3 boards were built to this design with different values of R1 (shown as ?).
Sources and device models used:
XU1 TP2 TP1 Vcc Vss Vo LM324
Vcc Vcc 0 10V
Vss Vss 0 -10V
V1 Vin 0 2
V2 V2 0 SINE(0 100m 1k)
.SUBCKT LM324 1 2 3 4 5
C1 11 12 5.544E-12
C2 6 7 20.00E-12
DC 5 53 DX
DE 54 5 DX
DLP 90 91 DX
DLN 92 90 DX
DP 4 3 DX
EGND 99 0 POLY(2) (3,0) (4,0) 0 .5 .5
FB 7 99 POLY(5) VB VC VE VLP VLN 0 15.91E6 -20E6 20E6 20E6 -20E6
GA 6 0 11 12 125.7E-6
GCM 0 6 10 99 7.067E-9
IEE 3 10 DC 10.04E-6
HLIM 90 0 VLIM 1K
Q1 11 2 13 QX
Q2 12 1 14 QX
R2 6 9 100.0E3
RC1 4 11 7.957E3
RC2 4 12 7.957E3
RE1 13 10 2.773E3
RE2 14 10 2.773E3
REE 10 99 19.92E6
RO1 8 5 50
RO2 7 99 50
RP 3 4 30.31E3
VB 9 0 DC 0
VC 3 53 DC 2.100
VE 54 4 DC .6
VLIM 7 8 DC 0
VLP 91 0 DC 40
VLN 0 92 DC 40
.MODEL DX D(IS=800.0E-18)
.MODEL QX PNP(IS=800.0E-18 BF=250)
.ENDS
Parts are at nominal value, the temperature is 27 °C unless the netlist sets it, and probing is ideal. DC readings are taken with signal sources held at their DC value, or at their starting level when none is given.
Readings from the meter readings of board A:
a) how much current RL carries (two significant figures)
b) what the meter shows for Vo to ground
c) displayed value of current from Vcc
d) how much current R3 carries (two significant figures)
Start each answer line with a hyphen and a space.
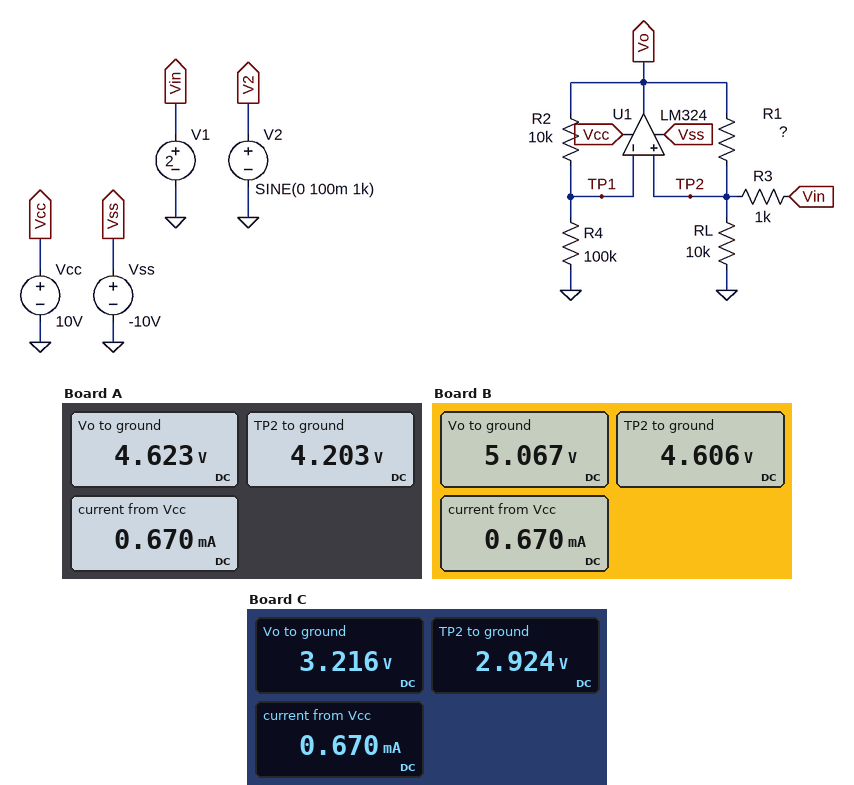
- 420 µA
- 4.623 V
- 0.670 mA
- 2.2 mA
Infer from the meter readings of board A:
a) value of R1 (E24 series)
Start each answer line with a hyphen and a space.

- 160 Ω
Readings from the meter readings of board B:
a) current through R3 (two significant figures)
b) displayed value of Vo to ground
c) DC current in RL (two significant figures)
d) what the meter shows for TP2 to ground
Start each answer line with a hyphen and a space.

- 2.6 mA
- 5.067 V
- 460 µA
- 4.606 V
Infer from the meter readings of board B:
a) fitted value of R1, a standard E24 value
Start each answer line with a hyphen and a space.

- 150 Ω
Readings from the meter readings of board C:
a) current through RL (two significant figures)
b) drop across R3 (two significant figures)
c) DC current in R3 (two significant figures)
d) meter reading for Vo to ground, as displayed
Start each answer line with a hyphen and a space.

- 290 µA
- 920 mV
- 920 µA
- 3.216 V
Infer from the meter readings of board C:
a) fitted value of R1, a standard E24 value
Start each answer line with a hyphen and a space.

- 240 Ω
